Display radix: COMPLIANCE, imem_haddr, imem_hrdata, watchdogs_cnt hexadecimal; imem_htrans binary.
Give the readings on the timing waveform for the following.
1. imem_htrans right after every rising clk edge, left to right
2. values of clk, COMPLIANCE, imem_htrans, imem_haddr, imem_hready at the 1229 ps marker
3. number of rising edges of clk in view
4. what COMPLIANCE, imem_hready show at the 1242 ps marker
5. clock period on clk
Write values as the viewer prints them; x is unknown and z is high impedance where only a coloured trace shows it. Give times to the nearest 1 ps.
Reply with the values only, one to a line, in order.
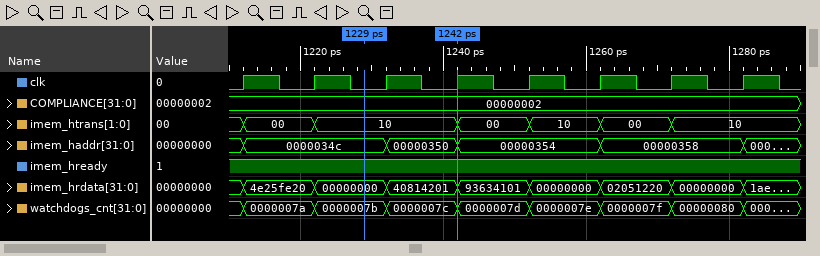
00, 10, 10, 00, 10, 00, 10, 10
clk=0, COMPLIANCE=00000002, imem_htrans=10, imem_haddr=0000034c, imem_hready=1
8
COMPLIANCE=00000002, imem_hready=1
10 ps
